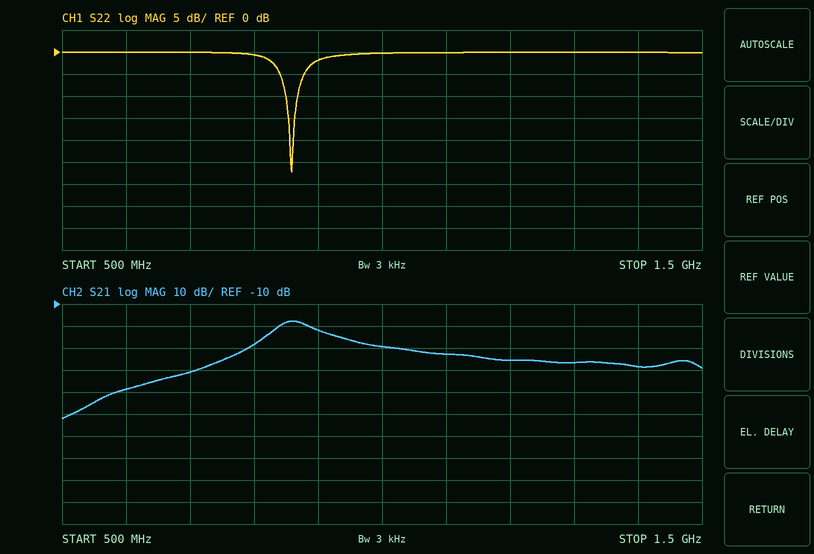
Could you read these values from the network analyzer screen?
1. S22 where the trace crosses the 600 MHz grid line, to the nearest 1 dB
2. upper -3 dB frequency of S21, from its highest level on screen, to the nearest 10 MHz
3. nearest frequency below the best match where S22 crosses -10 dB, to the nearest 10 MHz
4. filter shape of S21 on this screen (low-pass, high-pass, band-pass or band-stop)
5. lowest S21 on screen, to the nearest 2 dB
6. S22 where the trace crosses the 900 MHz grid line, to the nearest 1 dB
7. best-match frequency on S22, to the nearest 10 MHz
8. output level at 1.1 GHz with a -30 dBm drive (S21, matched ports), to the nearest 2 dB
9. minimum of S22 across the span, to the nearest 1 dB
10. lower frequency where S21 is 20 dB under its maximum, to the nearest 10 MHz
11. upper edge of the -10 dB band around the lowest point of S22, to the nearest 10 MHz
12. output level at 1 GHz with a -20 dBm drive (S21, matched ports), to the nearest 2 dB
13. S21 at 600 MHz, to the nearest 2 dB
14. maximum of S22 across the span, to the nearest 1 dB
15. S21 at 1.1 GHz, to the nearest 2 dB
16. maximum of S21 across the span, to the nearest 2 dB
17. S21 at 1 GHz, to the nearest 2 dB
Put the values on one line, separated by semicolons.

0 dB; 890 MHz; 850 MHz; band-pass; -62 dB; -2 dB; 860 MHz; -62 dBm; -27 dB; 730 MHz; 870 MHz; -50 dBm; -48 dB; 0 dB; -32 dB; -18 dB; -30 dB
